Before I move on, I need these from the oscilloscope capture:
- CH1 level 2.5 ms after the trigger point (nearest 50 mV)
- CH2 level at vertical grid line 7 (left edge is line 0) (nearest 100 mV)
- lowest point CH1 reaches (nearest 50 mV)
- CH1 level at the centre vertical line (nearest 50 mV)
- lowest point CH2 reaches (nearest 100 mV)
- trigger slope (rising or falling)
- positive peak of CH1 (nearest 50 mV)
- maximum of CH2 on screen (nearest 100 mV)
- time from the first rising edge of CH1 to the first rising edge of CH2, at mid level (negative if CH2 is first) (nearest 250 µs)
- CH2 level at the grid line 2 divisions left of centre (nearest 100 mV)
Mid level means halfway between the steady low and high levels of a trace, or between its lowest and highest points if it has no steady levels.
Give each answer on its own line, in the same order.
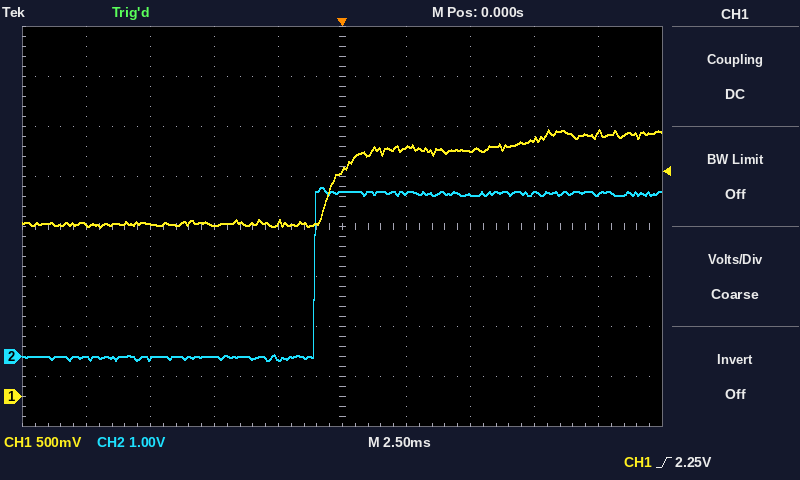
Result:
2.50 V
3.2 V
1.70 V
2.25 V
-100 mV
rising
2.65 V
3.4 V
-750 µs
0.0 V
